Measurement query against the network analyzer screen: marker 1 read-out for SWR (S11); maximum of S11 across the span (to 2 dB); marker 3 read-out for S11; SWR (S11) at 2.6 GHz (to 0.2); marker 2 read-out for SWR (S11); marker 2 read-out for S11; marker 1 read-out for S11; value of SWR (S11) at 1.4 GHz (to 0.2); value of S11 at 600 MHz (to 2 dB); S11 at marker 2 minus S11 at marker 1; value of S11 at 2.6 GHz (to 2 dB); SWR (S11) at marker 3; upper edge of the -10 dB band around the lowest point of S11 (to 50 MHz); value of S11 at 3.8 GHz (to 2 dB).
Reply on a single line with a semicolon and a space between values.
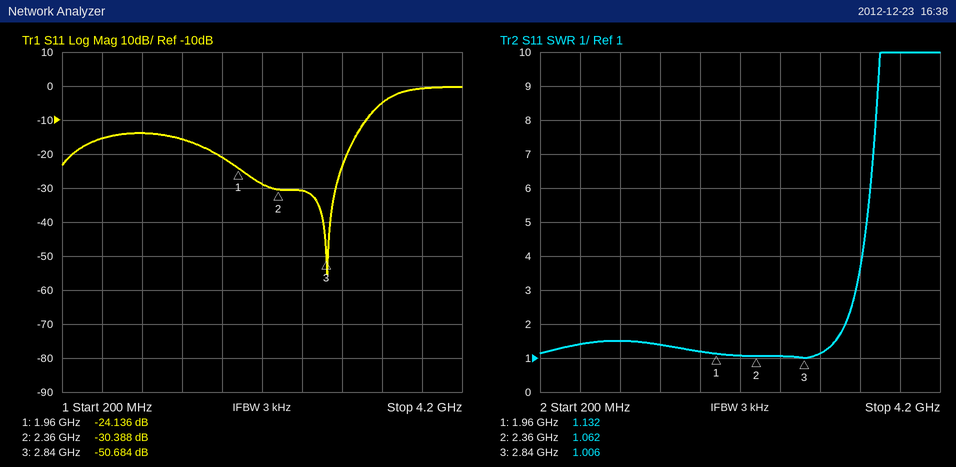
1.132; 0 dB; -50.684 dB; 1.0; 1.062; -30.388 dB; -24.136 dB; 1.4; -16 dB; -6.252 dB; -30 dB; 1.006; 3.25 GHz; 0 dB
